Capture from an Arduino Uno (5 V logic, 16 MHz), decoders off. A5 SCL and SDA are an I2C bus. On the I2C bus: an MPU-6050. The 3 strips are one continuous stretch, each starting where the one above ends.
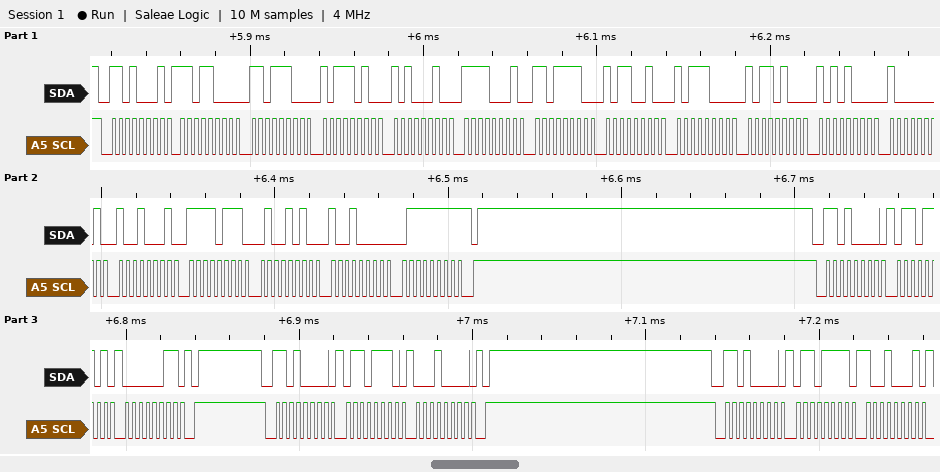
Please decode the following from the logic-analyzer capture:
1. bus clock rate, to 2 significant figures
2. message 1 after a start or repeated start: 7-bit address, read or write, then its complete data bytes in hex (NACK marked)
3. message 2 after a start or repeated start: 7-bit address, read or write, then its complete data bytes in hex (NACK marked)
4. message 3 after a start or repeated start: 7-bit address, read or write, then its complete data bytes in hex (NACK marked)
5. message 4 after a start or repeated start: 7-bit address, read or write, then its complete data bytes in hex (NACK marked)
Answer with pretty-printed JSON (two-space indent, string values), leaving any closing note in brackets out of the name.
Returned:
{
  "bus clock rate, to 2 significant figures": "250 kHz",
  "message 1 after a start or repeated start: 7-bit address, read or write, then its complete data bytes in hex": "0x68 read: D8 DC BA A2 F1 DE B2 B8 B4 A8 81 91 F7 4A 90 7F NACK",
  "message 2 after a start or repeated start: 7-bit address, read or write, then its complete data bytes in hex": "0x68 write: 6D 03",
  "message 3 after a start or repeated start: 7-bit address, read or write, then its complete data bytes in hex": "0x68 write: 6E 10",
  "message 4 after a start or repeated start: 7-bit address, read or write, then its complete data bytes in hex": "0x68 write: 6F 91"
}
